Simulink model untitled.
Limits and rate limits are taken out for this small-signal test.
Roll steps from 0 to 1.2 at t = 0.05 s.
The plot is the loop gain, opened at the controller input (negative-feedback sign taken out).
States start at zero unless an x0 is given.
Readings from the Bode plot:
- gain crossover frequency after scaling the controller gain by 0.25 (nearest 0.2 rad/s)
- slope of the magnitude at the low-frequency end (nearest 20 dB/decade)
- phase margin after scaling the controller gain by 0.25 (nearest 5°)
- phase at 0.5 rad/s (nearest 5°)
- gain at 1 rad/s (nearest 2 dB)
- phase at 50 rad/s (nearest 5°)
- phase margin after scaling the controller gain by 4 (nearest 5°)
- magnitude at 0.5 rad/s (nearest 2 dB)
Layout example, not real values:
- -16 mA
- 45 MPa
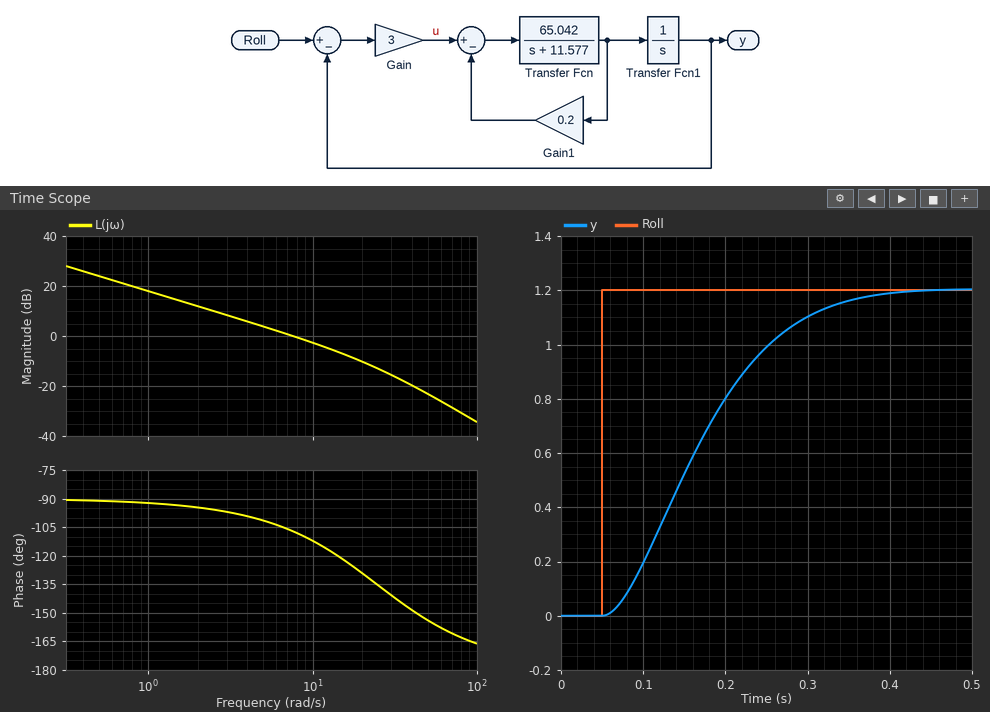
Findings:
- 2.0 rad/s
- -20 dB/decade
- 85°
- -90°
- 18 dB
- -155°
- 45°
- 24 dB
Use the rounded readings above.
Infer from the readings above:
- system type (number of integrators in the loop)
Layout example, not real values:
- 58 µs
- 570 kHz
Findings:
- 1
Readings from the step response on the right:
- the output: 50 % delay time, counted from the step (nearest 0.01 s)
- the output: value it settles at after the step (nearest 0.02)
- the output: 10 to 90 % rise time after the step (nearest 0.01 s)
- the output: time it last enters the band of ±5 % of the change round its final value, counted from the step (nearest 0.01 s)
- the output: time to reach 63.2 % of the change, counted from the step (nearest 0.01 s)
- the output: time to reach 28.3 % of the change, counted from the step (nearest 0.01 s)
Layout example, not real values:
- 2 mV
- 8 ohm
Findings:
- 0.11 s
- 1.20
- 0.20 s
- 0.28 s
- 0.14 s
- 0.07 s
